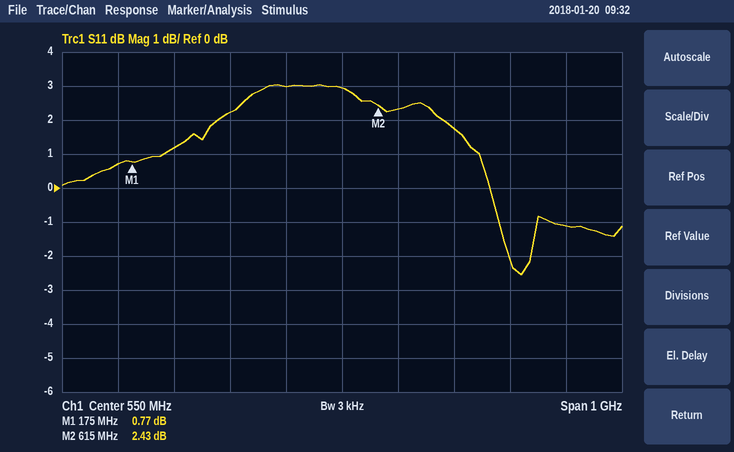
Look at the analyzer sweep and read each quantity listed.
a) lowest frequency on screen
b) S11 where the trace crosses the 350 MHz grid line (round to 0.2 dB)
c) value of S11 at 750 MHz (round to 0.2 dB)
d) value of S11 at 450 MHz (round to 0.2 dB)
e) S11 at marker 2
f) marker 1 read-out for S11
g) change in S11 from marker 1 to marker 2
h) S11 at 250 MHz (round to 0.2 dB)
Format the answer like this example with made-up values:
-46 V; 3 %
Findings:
50 MHz; 2.2 dB; 1.8 dB; 3.0 dB; 2.43 dB; 0.77 dB; 1.66 dB; 1.2 dB
